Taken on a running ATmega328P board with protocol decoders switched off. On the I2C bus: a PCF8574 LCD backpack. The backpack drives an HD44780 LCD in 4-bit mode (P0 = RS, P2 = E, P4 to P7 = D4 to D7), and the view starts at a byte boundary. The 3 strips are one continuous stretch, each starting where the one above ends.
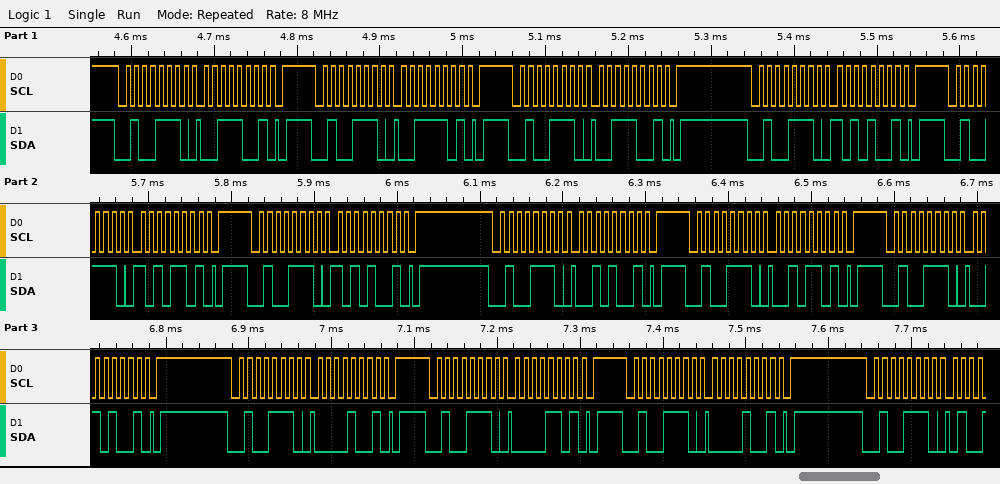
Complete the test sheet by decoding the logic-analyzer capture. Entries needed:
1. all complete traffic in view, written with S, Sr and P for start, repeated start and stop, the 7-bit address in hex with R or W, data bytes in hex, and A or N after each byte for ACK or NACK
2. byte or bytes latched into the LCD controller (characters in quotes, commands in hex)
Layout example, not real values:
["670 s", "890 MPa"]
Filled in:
["S 27W A 39 A P S 27W A 3D A P S 27W A 39 A P S 27W A A9 A P S 27W A AD A P S 27W A A9 A P S 27W A 29 A P S 27W A 2D A P S 27W A 29 A P S 27W A 09 A P S 27W A 0D A P S 27W A 09 A P S 27W A", "':' ' '"]
